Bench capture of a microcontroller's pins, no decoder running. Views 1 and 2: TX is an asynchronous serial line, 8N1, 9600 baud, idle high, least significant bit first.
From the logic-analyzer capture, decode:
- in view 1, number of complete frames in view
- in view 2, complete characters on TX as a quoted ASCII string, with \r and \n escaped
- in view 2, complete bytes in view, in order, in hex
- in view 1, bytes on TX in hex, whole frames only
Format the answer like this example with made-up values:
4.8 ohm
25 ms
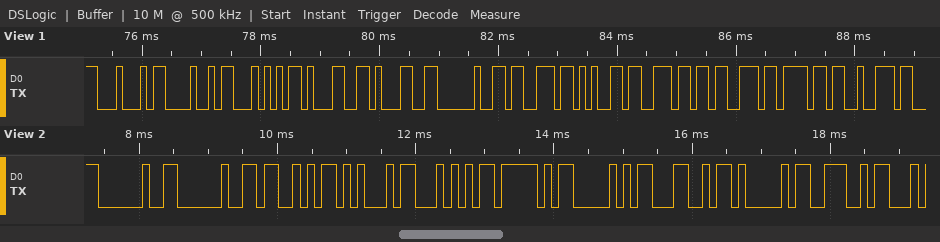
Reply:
12
"  SET_PLAN"
20 20 53 45 54 5F 50 4C 41 4E
44 48 54 31 31 20 73 65 6E 73 6F 72
